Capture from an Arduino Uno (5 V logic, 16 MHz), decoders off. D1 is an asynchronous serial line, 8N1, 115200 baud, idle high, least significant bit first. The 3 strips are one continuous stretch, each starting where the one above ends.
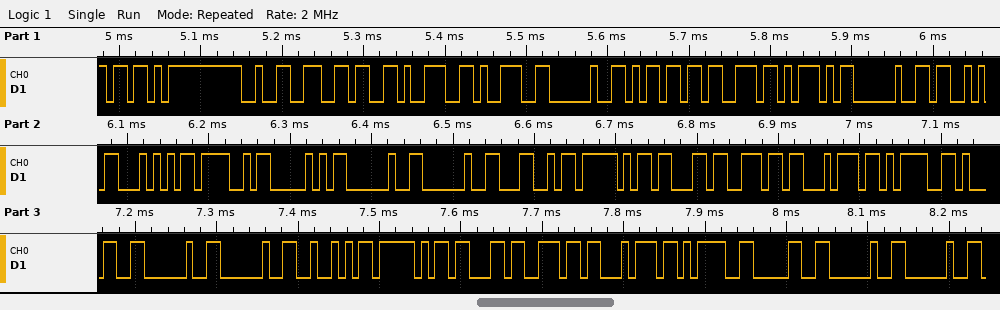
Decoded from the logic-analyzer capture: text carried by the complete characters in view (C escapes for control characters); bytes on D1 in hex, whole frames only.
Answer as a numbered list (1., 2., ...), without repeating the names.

1. "[2699 ms] STOP  L_cnt=1  R_cnt=0  "
2. 5B 32 36 39 39 20 6D 73 5D 20 53 54 4F 50 20 20 4C 5F 63 6E 74 3D 31 20 20 52 5F 63 6E 74 3D 30 20 20
